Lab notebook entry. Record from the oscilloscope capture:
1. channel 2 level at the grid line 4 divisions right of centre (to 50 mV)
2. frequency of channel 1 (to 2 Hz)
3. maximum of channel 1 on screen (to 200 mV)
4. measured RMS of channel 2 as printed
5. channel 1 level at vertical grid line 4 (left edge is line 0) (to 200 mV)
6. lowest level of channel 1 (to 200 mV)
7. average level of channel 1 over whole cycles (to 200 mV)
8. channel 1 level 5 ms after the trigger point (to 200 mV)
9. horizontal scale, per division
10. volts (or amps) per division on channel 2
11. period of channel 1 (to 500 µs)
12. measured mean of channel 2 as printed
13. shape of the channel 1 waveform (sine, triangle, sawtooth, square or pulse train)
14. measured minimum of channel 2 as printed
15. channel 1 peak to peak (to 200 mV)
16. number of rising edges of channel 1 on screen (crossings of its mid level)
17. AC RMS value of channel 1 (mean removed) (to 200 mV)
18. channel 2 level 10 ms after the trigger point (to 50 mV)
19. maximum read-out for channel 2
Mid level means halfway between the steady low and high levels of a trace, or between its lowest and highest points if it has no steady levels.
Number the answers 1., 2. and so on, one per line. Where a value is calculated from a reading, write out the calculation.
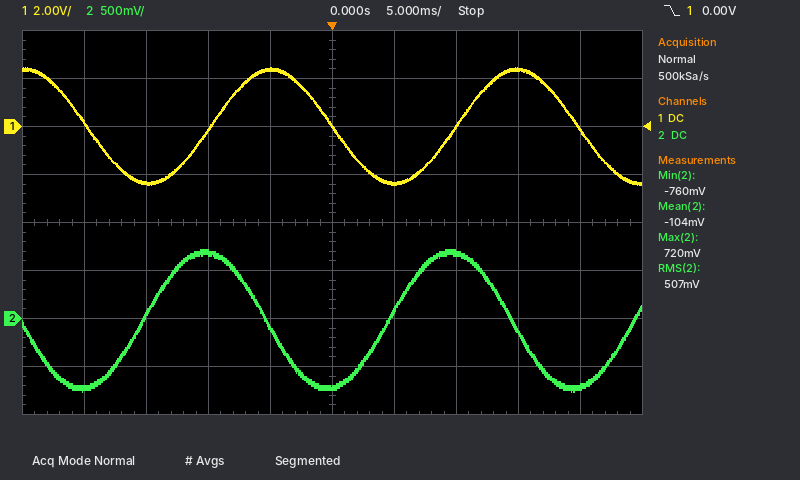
1. -700 mV
2. 1 / 20.0 ms ≈ 50 Hz
3. 2.4 V
4. 507 mV
5. 2.4 V
6. -2.4 V
7. (2.4 V + (-2.4 V)) / 2 ≈ 0.0 V
8. -2.4 V
9. 5 ms
10. 500 mV
11. 20.0 ms
12. -104 mV
13. sine
14. -760 mV
15. 2.4 V − (-2.4 V) = 4.8 V
16. 2
17. 4.8 V / (2√2) ≈ 1.70 V, so 1.6 V to the nearest 200 mV
18. 700 mV
19. 720 mV
